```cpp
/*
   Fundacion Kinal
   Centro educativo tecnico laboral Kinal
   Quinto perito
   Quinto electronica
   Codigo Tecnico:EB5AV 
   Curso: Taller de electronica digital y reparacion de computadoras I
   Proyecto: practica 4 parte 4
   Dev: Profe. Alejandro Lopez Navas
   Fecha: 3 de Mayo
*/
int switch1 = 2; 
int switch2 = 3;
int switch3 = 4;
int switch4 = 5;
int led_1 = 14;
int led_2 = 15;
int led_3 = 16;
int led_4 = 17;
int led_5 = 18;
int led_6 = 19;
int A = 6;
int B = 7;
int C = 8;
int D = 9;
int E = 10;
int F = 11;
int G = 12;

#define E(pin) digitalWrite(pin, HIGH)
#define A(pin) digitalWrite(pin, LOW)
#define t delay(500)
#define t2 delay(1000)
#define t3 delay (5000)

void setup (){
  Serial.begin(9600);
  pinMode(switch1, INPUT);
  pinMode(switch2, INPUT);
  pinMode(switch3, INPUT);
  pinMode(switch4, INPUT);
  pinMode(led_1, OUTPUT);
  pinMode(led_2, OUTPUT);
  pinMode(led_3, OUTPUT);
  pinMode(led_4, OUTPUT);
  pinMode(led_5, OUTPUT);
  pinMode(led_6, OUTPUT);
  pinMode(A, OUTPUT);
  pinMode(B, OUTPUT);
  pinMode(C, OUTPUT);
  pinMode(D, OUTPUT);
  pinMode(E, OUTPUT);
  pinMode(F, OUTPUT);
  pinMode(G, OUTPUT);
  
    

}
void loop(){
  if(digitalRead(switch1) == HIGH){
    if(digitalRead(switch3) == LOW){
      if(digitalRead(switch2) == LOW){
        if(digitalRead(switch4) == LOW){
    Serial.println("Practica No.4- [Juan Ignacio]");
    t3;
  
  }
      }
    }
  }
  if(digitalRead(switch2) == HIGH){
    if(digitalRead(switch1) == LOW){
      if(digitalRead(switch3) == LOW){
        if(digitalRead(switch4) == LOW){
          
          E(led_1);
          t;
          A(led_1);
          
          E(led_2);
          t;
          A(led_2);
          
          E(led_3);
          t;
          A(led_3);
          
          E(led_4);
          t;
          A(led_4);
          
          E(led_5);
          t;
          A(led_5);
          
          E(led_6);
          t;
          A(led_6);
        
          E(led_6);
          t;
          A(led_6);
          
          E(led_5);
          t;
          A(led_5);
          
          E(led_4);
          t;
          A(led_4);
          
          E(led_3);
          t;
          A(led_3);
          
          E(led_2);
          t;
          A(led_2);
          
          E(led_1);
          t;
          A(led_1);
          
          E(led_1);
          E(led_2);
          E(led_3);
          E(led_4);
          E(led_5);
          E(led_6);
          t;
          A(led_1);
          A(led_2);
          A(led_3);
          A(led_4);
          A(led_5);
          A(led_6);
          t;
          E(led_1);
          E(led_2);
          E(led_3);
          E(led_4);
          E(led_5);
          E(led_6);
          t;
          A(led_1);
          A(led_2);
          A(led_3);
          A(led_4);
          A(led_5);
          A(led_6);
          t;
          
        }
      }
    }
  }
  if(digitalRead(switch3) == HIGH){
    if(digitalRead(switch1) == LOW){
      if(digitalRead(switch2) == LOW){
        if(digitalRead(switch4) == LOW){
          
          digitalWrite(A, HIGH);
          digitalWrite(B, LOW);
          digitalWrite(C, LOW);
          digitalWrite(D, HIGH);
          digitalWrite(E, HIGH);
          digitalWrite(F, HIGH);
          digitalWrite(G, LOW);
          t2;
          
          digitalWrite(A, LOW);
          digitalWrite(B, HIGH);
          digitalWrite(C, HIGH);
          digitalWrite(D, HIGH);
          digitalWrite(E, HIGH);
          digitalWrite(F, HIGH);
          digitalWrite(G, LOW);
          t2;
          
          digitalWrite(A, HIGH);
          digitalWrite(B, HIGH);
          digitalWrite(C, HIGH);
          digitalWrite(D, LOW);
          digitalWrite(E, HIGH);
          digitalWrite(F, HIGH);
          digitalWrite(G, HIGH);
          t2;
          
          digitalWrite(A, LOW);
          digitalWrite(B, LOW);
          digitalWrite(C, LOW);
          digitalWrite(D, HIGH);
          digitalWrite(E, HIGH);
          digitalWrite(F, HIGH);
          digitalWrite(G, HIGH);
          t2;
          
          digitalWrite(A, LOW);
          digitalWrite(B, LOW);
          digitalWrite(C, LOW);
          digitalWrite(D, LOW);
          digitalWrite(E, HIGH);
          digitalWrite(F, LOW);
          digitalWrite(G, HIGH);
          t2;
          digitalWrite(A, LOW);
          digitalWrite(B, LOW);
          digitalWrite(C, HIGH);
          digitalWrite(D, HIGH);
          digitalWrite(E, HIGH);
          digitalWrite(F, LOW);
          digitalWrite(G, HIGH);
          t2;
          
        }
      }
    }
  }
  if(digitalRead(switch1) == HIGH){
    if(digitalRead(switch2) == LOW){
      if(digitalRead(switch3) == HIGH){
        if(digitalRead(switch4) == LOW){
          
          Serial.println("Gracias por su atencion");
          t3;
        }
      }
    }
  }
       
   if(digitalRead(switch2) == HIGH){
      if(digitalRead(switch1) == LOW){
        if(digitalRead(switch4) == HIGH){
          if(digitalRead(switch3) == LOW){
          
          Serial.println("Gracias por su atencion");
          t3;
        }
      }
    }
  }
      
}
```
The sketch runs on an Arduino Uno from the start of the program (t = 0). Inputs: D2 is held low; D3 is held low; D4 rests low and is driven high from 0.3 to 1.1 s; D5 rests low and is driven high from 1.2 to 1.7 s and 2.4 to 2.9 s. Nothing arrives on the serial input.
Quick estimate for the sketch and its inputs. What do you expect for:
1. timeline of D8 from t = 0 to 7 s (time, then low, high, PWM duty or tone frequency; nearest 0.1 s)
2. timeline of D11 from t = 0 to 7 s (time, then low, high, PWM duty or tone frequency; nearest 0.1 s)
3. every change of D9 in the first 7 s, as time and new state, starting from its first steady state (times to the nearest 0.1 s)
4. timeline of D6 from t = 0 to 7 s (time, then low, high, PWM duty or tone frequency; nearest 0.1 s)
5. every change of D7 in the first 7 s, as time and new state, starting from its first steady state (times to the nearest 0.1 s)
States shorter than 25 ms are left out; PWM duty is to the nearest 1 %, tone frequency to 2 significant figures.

0 s low; 1.3 s high; 3.3 s low; 5.3 s high
0 s low; 0.3 s high; 4.3 s low
0 s low; 0.3 s high; 2.3 s low; 3.3 s high; 4.3 s low; 5.3 s high
0 s low; 0.3 s high; 1.3 s low; 2.3 s high; 3.3 s low
0 s low; 1.3 s high; 3.3 s low
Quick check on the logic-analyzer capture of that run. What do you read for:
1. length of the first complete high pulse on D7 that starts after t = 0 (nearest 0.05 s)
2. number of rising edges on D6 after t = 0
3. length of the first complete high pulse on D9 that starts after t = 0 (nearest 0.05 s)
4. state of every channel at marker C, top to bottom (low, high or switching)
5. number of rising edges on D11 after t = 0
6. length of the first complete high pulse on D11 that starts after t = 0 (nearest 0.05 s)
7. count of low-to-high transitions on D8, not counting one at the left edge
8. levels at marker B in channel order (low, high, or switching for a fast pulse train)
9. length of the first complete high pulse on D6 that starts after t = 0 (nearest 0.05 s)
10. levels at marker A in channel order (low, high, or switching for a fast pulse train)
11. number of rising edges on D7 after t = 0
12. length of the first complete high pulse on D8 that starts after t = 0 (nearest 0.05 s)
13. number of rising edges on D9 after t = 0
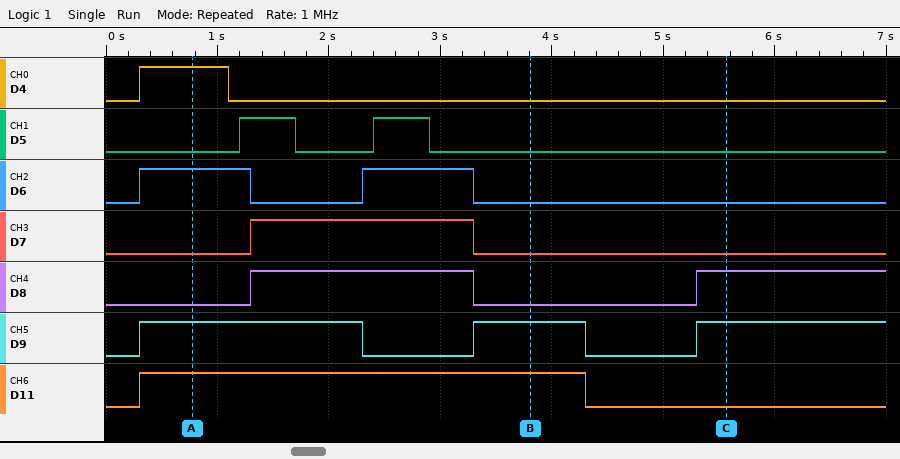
2.00 s
2
2.00 s
D4 low, D5 low, D6 low, D7 low, D8 high, D9 high, D11 low
1
4.00 s
2
D4 low, D5 low, D6 low, D7 low, D8 low, D9 high, D11 high
1.00 s
D4 high, D5 low, D6 high, D7 low, D8 low, D9 high, D11 high
1
2.00 s
3
